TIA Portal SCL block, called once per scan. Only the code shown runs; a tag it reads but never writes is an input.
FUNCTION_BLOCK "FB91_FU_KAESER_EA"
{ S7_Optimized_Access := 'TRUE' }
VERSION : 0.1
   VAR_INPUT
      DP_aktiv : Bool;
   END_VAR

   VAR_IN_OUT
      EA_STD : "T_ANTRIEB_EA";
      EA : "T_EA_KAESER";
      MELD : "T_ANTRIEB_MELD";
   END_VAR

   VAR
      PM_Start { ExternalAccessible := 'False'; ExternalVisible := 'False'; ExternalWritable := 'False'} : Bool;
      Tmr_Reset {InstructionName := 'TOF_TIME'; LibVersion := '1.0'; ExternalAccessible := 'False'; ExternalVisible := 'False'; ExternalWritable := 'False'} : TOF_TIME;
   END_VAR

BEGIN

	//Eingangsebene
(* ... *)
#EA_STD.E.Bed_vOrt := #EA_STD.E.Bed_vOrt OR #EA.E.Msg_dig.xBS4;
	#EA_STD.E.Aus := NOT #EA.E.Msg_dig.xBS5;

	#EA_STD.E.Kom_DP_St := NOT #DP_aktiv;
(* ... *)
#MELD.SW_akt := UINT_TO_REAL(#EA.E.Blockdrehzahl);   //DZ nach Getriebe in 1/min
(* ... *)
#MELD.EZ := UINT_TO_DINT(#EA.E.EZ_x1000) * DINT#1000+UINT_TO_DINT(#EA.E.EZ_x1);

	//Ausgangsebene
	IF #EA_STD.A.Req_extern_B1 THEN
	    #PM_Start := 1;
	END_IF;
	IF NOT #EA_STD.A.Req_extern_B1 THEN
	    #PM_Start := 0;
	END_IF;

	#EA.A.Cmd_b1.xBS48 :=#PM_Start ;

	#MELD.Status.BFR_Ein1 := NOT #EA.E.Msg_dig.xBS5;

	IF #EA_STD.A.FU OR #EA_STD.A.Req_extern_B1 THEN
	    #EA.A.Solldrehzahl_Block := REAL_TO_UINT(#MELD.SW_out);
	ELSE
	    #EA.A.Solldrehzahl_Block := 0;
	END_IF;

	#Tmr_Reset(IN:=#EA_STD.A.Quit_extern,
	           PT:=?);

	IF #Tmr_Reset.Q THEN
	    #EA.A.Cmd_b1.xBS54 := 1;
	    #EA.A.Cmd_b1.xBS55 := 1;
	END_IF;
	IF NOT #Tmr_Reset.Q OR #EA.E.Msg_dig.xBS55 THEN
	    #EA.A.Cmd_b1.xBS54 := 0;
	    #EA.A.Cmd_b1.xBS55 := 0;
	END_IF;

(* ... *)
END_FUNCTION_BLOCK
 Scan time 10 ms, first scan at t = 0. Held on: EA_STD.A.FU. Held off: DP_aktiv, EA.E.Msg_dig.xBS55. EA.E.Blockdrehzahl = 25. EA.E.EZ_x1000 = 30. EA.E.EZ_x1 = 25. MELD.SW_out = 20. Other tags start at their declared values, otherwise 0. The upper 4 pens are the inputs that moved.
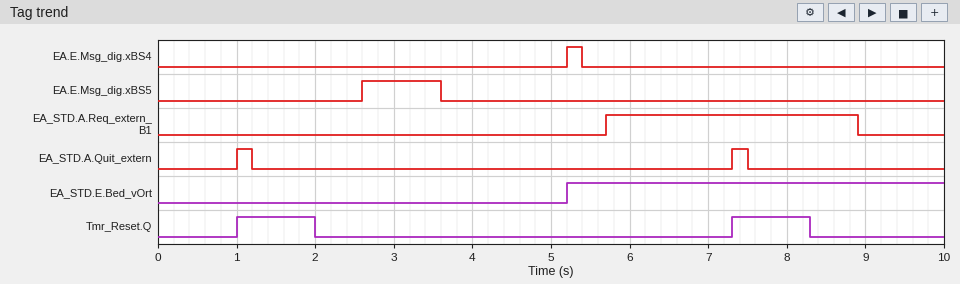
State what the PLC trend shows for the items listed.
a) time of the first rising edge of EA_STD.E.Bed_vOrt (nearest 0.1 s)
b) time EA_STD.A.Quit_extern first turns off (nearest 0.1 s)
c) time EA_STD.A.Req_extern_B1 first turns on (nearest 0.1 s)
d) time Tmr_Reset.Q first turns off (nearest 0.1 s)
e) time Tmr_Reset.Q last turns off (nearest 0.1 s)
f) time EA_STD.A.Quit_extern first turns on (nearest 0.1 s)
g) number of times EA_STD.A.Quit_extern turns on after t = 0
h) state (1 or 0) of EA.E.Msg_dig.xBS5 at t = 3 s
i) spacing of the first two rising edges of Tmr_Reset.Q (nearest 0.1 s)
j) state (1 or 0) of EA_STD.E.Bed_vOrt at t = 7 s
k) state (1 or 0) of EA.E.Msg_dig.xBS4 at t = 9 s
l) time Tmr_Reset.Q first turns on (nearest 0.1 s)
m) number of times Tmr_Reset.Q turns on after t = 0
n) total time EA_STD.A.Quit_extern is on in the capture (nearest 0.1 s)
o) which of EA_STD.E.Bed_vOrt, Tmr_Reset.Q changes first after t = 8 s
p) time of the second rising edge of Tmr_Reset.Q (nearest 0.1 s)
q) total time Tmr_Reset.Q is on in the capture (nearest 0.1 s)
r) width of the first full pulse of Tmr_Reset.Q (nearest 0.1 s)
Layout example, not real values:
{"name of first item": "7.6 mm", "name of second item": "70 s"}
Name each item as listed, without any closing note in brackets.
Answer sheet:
{"time of the first rising edge of EA_STD.E.Bed_vOrt": "5.2 s", "time EA_STD.A.Quit_extern first turns off": "1.2 s", "time EA_STD.A.Req_extern_B1 first turns on": "5.7 s", "time Tmr_Reset.Q first turns off": "2.0 s", "time Tmr_Reset.Q last turns off": "8.3 s", "time EA_STD.A.Quit_extern first turns on": "1.0 s", "number of times EA_STD.A.Quit_extern turns on after t = 0": "2", "state (1 or 0) of EA.E.Msg_dig.xBS5 at t = 3 s": "1", "spacing of the first two rising edges of Tmr_Reset.Q": "6.3 s", "state (1 or 0) of EA_STD.E.Bed_vOrt at t = 7 s": "1", "state (1 or 0) of EA.E.Msg_dig.xBS4 at t = 9 s": "0", "time Tmr_Reset.Q first turns on": "1.0 s", "number of times Tmr_Reset.Q turns on after t = 0": "2", "total time EA_STD.A.Quit_extern is on in the capture": "0.4 s", "which of EA_STD.E.Bed_vOrt, Tmr_Reset.Q changes first after t = 8 s": "Tmr_Reset.Q", "time of the second rising edge of Tmr_Reset.Q": "7.3 s", "total time Tmr_Reset.Q is on in the capture": "2.0 s", "width of the first full pulse of Tmr_Reset.Q": "1.0 s"}
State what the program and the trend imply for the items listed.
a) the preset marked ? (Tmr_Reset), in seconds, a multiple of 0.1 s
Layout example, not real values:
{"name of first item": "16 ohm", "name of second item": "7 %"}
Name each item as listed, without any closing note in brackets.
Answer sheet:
{"the preset marked ? (Tmr_Reset), in seconds, a multiple of 0.1 s": "0.8 s"}
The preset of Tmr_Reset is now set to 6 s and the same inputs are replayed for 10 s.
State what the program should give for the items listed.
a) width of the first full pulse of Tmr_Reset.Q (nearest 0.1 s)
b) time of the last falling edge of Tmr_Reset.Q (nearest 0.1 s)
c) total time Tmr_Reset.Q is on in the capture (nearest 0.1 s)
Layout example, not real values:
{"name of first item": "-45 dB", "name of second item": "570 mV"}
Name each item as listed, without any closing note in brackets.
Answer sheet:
{"width of the first full pulse of Tmr_Reset.Q": "6.2 s", "time of the last falling edge of Tmr_Reset.Q": "7.2 s", "total time Tmr_Reset.Q is on in the capture": "8.9 s"}
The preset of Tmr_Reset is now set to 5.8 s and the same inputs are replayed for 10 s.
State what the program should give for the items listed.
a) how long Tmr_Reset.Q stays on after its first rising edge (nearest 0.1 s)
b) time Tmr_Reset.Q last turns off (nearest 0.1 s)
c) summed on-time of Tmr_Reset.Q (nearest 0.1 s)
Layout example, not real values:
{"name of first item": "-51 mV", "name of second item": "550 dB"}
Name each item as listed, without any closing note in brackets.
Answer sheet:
{"how long Tmr_Reset.Q stays on after its first rising edge": "6.0 s", "time Tmr_Reset.Q last turns off": "7.0 s", "summed on-time of Tmr_Reset.Q": "8.7 s"}
